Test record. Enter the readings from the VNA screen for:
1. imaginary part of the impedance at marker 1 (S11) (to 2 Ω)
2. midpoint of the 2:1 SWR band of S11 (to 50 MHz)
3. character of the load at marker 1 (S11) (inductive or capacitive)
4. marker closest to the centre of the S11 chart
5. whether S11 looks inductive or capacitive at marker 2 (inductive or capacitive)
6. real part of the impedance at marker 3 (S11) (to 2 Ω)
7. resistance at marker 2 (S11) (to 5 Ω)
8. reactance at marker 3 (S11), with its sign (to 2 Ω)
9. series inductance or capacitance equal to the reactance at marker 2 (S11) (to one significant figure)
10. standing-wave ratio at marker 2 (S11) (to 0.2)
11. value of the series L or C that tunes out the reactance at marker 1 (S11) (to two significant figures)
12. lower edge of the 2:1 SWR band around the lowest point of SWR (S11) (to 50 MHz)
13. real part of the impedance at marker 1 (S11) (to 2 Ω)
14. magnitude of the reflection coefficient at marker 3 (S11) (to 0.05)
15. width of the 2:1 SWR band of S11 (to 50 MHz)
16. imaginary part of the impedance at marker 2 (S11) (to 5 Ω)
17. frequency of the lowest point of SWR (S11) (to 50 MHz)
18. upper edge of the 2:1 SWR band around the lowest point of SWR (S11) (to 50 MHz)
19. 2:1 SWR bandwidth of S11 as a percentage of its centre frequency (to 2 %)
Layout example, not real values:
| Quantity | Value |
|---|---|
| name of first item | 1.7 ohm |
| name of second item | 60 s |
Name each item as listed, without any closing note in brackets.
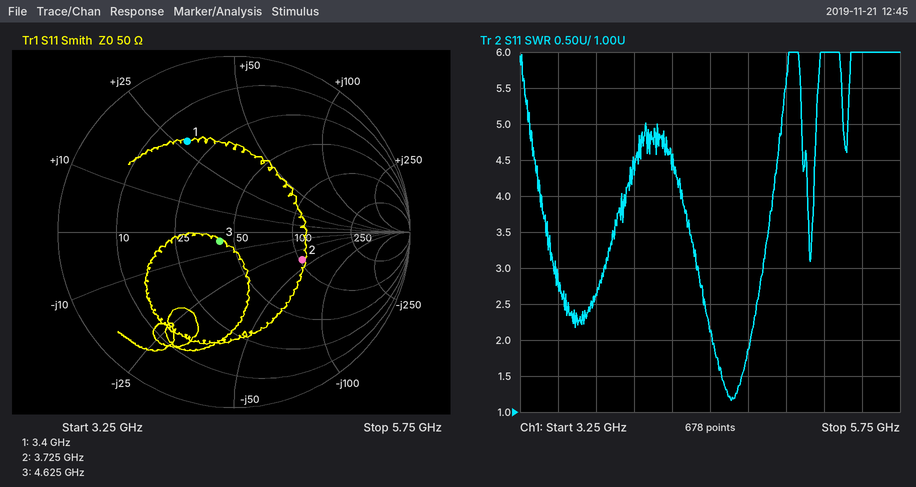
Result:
| Quantity | Value |
|---|---|
| imaginary part of the impedance at marker 1 (S11) | +28 Ω |
| midpoint of the 2:1 SWR band of S11 | 4.65 GHz |
| character of the load at marker 1 (S11) | inductive |
| marker closest to the centre of the S11 chart | marker 3 |
| whether S11 looks inductive or capacitive at marker 2 | capacitive |
| real part of the impedance at marker 3 (S11) | 42 Ω |
| resistance at marker 2 (S11) | 105 Ω |
| reactance at marker 3 (S11), with its sign | -4 Ω |
| series inductance or capacitance equal to the reactance at marker 2 (S11) | 1 pF |
| standing-wave ratio at marker 2 (S11) | 2.4 |
| value of the series L or C that tunes out the reactance at marker 1 (S11) | 1.7 pF |
| lower edge of the 2:1 SWR band around the lowest point of SWR (S11) | 4.50 GHz |
| real part of the impedance at marker 1 (S11) | 18 Ω |
| magnitude of the reflection coefficient at marker 3 (S11) | 0.10 |
| width of the 2:1 SWR band of S11 | 250 MHz |
| imaginary part of the impedance at marker 2 (S11) | -40 Ω |
| frequency of the lowest point of SWR (S11) | 4.65 GHz |
| upper edge of the 2:1 SWR band around the lowest point of SWR (S11) | 4.75 GHz |
| 2:1 SWR bandwidth of S11 as a percentage of its centre frequency | 6 % |
